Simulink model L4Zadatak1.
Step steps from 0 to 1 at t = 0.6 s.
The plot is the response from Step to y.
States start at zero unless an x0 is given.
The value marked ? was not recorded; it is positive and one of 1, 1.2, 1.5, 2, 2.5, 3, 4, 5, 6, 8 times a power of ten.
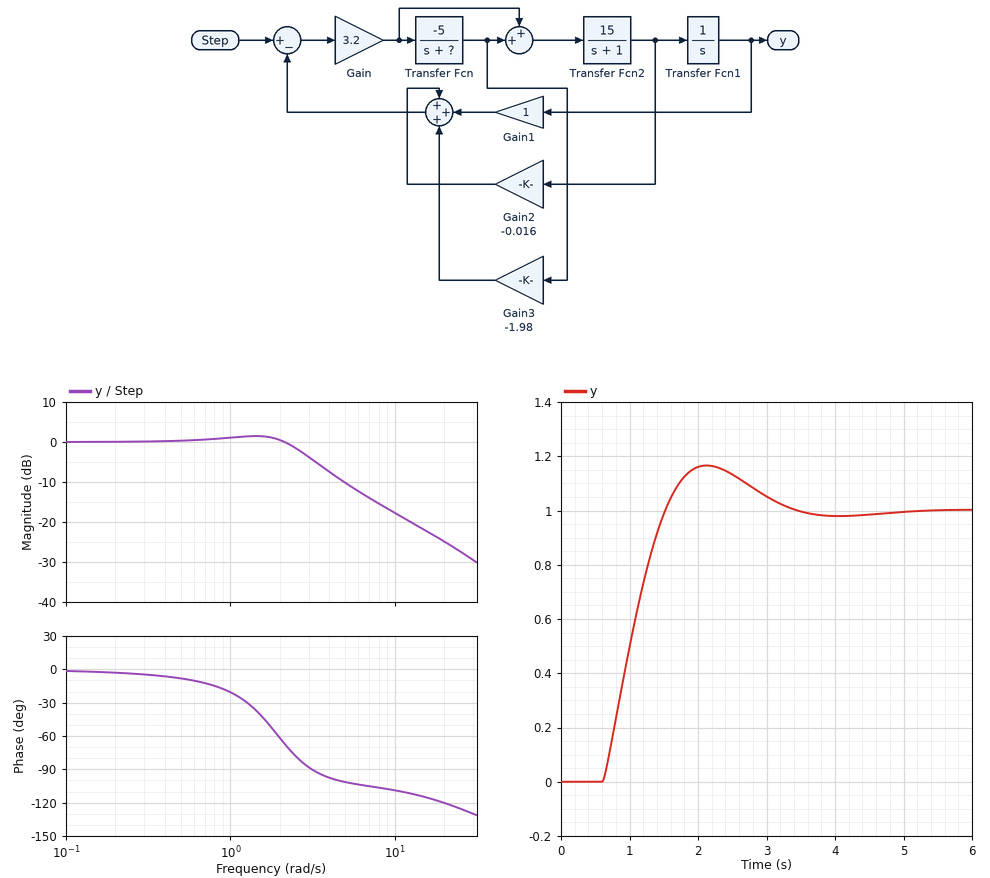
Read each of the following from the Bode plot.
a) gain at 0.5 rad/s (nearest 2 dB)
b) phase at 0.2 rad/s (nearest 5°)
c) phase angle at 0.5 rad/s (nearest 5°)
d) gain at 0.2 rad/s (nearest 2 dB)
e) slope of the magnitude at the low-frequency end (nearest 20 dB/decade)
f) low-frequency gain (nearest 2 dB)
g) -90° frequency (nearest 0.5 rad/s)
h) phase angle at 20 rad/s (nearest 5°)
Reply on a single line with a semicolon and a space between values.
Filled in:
0 dB; -5°; -10°; 0 dB; 0 dB/decade; 0 dB; 3.0 rad/s; -120°
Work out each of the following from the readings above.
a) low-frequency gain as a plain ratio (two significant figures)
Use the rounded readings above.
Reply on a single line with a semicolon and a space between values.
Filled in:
1.0
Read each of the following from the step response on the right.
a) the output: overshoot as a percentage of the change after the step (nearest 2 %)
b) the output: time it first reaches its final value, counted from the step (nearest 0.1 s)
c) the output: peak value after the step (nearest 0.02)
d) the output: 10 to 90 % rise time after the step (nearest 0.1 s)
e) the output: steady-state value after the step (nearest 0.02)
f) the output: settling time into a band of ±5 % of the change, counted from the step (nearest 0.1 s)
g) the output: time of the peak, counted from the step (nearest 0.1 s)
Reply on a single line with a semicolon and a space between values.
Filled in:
16 %; 0.9 s; 1.16; 0.7 s; 1.00; 2.4 s; 1.5 s
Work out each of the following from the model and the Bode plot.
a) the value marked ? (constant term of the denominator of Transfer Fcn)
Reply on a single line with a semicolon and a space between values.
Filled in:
8
